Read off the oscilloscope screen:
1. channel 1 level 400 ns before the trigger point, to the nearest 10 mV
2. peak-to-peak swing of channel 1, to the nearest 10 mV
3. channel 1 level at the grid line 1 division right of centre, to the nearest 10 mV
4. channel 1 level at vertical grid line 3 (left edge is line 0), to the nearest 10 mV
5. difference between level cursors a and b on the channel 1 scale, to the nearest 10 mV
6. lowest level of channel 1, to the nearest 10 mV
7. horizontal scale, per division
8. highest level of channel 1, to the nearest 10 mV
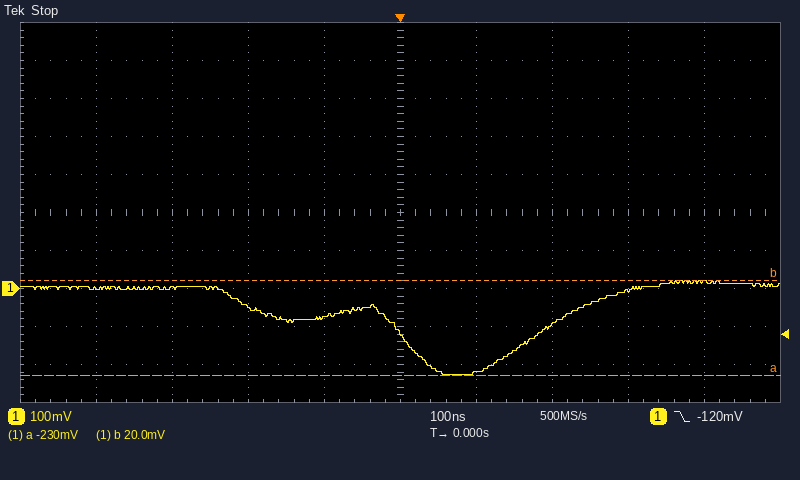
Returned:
0 mV
250 mV
-220 mV
-50 mV
250 mV
-230 mV
100 ns
20 mV
